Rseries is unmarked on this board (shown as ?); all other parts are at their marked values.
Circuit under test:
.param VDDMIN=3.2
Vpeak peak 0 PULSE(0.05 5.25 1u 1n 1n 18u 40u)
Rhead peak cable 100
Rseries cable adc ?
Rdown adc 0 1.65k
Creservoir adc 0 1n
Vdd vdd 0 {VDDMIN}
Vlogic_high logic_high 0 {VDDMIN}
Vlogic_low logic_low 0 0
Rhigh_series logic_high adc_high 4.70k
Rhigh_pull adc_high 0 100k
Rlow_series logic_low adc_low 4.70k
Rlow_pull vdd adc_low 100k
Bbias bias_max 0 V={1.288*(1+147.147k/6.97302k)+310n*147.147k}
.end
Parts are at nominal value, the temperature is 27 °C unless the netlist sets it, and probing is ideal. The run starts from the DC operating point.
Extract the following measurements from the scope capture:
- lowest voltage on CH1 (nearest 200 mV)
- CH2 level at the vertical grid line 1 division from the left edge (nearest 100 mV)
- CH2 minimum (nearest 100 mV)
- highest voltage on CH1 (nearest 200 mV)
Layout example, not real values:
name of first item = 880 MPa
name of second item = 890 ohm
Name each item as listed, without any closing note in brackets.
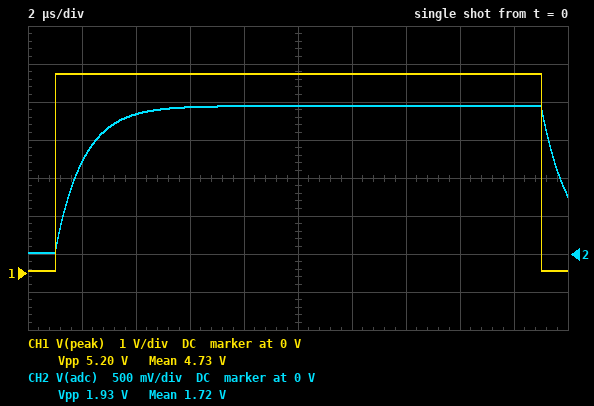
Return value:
lowest voltage on CH1 = 0 V
CH2 level at the vertical grid line 1 division from the left edge = 1.2 V
CH2 minimum = 0 V
highest voltage on CH1 = 5.2 V
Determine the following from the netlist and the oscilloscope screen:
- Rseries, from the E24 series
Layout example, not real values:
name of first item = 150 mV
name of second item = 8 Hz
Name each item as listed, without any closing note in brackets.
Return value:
Rseries, from the E24 series = 2.7 kΩ
